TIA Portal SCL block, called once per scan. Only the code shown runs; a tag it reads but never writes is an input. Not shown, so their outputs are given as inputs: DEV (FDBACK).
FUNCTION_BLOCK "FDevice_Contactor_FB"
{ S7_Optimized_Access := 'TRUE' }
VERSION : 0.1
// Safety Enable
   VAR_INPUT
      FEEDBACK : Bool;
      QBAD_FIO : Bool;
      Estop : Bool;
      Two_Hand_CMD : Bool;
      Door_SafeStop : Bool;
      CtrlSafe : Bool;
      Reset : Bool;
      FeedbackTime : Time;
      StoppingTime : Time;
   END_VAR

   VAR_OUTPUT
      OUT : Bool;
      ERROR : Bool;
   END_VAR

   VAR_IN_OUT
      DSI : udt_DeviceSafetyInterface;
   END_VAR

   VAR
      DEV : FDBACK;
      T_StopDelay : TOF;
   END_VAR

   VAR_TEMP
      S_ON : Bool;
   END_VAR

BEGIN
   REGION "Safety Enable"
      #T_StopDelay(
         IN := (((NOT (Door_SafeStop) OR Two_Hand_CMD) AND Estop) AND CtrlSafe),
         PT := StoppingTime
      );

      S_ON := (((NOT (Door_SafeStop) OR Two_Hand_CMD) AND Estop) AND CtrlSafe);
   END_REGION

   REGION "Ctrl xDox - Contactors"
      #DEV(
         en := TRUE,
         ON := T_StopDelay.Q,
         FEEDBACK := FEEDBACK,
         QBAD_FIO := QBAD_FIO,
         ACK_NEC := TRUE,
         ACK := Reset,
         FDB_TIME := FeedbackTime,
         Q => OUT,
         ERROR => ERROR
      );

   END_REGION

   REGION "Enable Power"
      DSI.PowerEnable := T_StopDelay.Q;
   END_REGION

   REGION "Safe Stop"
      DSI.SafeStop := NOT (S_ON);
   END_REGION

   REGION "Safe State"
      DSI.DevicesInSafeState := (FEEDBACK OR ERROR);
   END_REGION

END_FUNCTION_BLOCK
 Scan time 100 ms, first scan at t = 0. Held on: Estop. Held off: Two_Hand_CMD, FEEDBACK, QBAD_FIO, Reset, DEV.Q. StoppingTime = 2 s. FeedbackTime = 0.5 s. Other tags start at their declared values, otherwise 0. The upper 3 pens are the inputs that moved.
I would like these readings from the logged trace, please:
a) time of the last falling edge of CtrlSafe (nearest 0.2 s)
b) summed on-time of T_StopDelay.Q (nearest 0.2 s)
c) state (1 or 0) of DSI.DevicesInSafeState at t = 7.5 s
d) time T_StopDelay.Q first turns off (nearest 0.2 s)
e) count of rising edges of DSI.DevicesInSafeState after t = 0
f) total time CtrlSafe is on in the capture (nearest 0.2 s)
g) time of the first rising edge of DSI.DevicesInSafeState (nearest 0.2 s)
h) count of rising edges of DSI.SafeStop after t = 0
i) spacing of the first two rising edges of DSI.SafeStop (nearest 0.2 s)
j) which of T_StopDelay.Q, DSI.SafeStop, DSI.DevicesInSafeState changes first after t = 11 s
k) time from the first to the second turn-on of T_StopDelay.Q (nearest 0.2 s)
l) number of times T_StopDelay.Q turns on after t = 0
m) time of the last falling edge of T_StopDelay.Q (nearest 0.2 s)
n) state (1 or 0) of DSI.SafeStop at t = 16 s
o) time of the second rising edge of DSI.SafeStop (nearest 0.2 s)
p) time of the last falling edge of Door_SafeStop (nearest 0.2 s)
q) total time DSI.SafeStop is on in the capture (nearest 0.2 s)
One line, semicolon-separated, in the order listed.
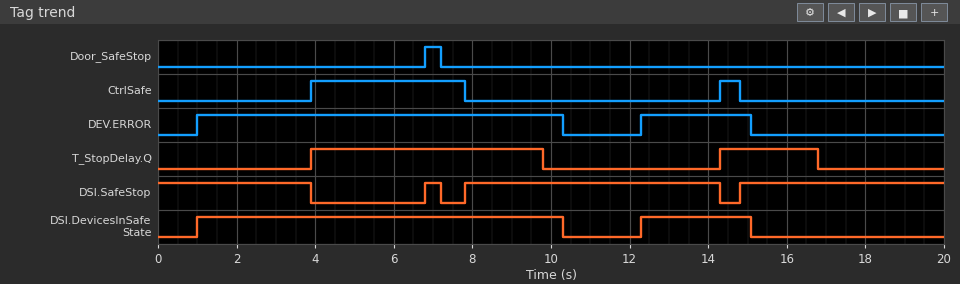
14.8 s; 8.4 s; 1; 9.8 s; 2; 4.4 s; 1.0 s; 3; 1.0 s; DSI.DevicesInSafeState; 10.4 s; 2; 16.8 s; 1; 7.8 s; 7.2 s; 16.0 s
